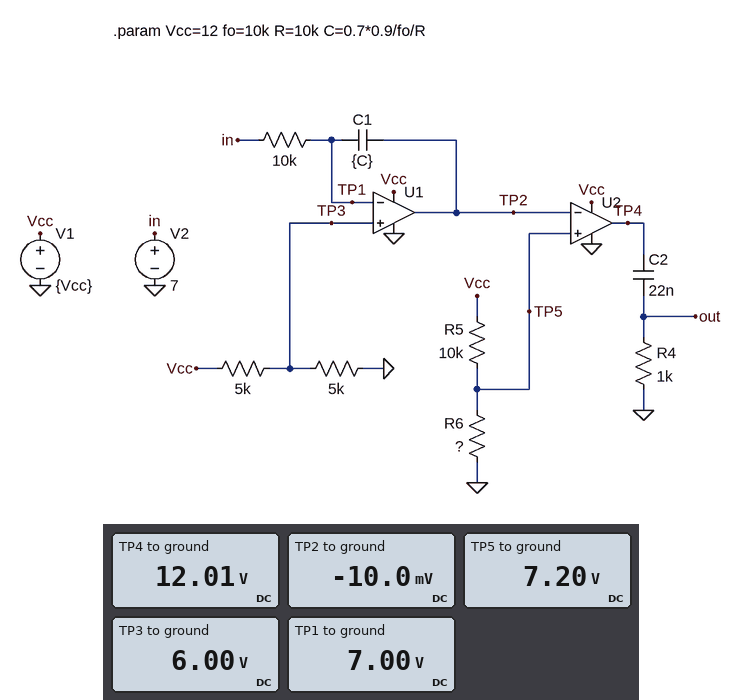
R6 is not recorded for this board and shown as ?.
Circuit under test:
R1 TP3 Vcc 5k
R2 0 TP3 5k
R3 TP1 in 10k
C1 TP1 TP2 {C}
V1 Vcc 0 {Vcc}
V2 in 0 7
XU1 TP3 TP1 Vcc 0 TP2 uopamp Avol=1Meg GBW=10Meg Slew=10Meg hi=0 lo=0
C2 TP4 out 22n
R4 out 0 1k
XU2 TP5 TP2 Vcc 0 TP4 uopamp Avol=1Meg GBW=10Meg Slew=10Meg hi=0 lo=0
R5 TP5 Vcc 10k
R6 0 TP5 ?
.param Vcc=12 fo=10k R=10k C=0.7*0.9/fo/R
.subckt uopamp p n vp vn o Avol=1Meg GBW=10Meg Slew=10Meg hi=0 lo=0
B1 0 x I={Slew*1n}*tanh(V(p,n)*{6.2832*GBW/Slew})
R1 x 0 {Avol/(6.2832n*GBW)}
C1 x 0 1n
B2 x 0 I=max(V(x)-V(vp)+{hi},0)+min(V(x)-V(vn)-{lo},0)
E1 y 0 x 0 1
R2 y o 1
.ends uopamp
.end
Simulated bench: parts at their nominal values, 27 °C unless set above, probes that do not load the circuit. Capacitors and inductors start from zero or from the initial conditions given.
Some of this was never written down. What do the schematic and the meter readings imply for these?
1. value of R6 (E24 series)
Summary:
15 kΩ
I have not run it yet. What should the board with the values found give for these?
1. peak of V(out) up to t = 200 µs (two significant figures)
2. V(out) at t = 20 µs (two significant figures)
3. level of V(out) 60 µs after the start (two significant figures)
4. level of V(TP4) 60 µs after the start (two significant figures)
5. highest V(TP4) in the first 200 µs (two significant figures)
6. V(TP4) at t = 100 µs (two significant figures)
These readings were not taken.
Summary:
12 V
5.0 V
810 mV
12 V
12 V
12 V
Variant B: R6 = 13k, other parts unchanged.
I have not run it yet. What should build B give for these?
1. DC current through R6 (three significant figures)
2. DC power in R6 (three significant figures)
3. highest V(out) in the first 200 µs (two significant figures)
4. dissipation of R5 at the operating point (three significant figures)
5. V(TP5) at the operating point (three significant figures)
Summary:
522 µA
3.54 mW
12 V
2.72 mW
6.78 V
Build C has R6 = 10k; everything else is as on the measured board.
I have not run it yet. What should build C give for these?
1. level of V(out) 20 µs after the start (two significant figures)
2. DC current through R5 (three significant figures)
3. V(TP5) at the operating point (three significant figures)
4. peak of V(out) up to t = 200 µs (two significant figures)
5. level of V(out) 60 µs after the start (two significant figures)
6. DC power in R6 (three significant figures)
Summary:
5.1 V
600 µA
6.00 V
11 V
820 mV
3.60 mW
